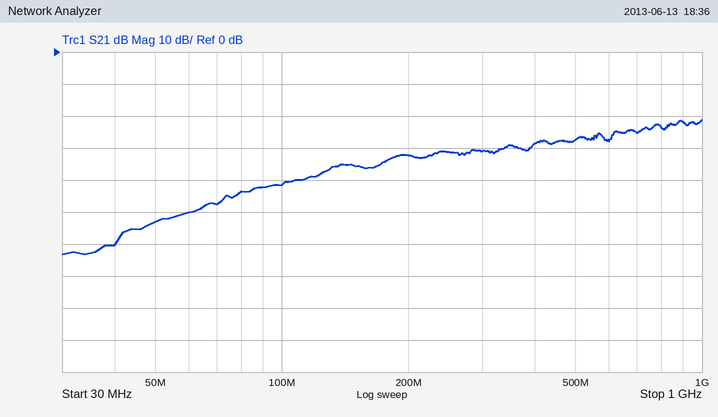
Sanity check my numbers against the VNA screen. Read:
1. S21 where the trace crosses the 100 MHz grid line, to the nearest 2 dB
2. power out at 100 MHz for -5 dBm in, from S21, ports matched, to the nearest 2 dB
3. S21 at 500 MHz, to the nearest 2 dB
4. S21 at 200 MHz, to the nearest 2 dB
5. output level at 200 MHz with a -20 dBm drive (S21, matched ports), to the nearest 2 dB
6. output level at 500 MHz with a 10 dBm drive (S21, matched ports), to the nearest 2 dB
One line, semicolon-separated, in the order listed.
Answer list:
-42 dB; -46 dBm; -28 dB; -32 dB; -52 dBm; -18 dBm
